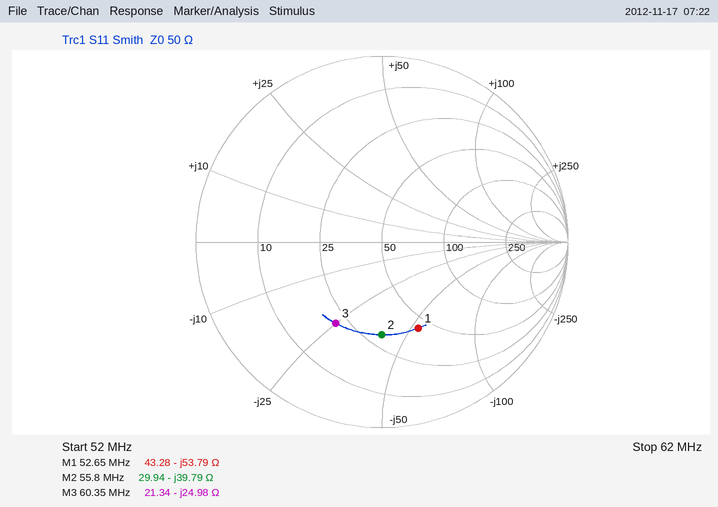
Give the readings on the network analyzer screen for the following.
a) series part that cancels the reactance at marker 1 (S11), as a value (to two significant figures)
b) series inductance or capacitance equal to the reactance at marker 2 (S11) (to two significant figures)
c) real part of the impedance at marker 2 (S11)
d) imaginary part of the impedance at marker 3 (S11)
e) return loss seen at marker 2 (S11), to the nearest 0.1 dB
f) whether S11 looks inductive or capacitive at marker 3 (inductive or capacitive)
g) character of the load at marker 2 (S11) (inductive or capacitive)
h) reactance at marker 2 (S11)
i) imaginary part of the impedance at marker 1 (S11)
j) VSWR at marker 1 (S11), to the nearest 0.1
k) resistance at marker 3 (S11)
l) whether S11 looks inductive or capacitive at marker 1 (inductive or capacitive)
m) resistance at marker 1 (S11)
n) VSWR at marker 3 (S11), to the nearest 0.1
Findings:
160 nH
72 pF
29.94 Ω
-24.98 Ω
6.0 dB
capacitive
capacitive
-39.79 Ω
-53.79 Ω
3.0
21.34 Ω
capacitive
43.28 Ω
3.0
